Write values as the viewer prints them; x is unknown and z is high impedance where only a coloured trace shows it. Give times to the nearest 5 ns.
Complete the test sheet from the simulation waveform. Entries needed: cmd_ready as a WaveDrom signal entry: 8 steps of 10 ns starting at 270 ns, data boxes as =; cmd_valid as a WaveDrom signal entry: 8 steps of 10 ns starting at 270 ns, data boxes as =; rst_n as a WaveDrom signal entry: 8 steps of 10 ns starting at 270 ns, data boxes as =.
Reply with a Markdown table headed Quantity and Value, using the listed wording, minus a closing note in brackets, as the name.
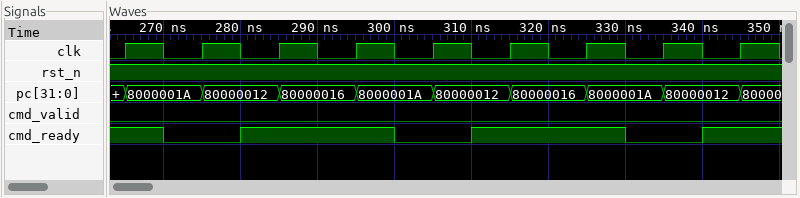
| Quantity | Value |
|---|---|
| cmd_ready as a WaveDrom signal entry: 8 steps of 10 ns starting at 270 ns, data boxes as = | {name: 'cmd_ready', wave: '01.01.01'} |
| cmd_valid as a WaveDrom signal entry: 8 steps of 10 ns starting at 270 ns, data boxes as = | {name: 'cmd_valid', wave: '0.......'} |
| rst_n as a WaveDrom signal entry: 8 steps of 10 ns starting at 270 ns, data boxes as = | {name: 'rst_n', wave: '1.......'} |
